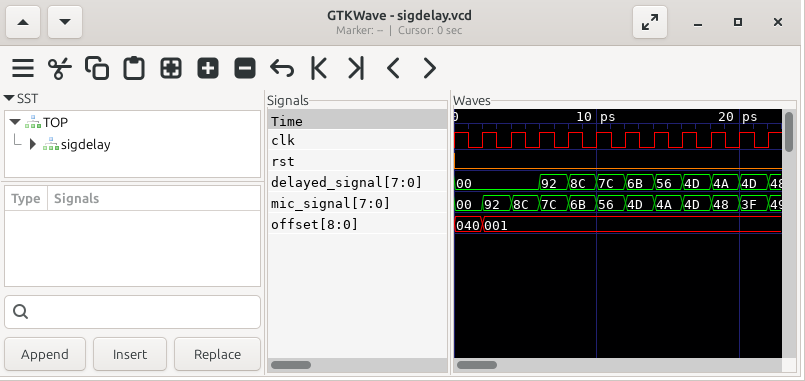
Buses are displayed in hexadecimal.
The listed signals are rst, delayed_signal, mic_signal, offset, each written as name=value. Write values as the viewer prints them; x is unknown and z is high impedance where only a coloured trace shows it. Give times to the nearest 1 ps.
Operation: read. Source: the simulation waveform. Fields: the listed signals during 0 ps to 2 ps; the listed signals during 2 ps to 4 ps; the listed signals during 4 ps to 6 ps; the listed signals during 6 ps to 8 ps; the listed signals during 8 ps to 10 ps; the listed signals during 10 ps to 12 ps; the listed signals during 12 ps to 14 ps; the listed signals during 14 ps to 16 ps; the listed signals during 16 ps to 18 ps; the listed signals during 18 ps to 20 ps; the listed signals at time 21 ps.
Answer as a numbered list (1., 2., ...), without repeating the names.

1. rst=0, delayed_signal=00, mic_signal=00, offset=040
2. rst=0, delayed_signal=00, mic_signal=92, offset=001
3. rst=0, delayed_signal=00, mic_signal=8C, offset=001
4. rst=0, delayed_signal=92, mic_signal=7C, offset=001
5. rst=0, delayed_signal=8C, mic_signal=6B, offset=001
6. rst=0, delayed_signal=7C, mic_signal=56, offset=001
7. rst=0, delayed_signal=6B, mic_signal=4D, offset=001
8. rst=0, delayed_signal=56, mic_signal=4A, offset=001
9. rst=0, delayed_signal=4D, mic_signal=4D, offset=001
10. rst=0, delayed_signal=4A, mic_signal=48, offset=001
11. rst=0, delayed_signal=4D, mic_signal=3F, offset=001
